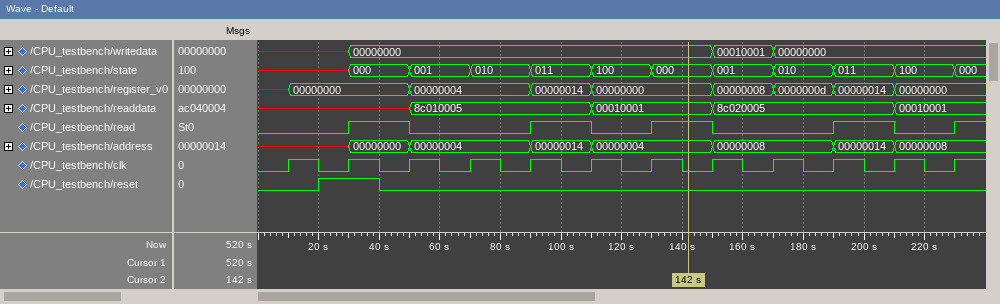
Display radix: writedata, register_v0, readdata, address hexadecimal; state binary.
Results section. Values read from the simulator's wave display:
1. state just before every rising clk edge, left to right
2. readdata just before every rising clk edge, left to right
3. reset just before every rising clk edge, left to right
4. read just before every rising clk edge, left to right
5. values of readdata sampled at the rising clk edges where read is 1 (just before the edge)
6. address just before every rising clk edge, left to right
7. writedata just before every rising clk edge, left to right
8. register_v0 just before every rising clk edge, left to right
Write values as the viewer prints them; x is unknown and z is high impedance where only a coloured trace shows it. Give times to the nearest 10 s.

x, x, 000, 001, 010, 011, 100, 000, 001, 010, 011, 100
x, x, x, 8c010005, 8c010005, 8c010005, 00010001, 00010001, 8c020005, 8c020005, 8c020005, 00010001
0 1 0 0 0 0 0 0 0 0 0 0
0 0 1 0 0 1 0 1 0 0 1 0
x, 8c010005, 00010001, 8c020005
x, x, 00000000, 00000004, 00000004, 00000014, 00000004, 00000004, 00000008, 00000008, 00000014, 00000008
x, x, 00000000, 00000000, 00000000, 00000000, 00000000, 00000000, 00010001, 00000000, 00000000, 00000000
x, 00000000, 00000000, 00000004, 00000004, 00000014, 00000000, 00000000, 00000008, 0000000d, 00000014, 00000000
